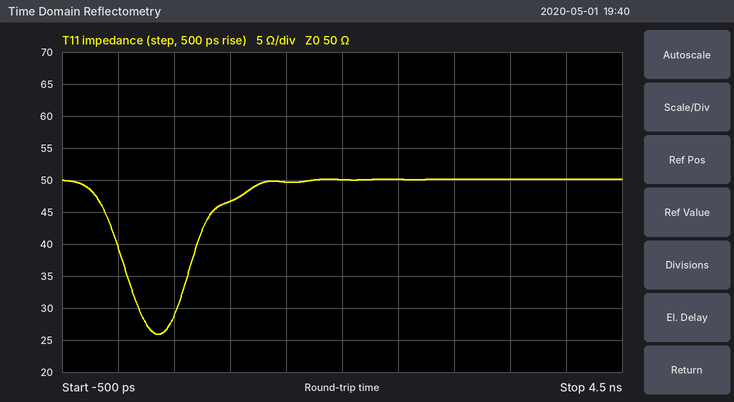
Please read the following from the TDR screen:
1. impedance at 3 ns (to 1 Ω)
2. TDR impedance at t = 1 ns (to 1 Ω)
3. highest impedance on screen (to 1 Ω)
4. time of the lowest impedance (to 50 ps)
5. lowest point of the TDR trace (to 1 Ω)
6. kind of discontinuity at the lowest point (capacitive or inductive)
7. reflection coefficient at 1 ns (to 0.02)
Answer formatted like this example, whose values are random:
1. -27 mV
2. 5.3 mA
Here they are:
1. 50 Ω
2. 47 Ω
3. 50 Ω
4. 350 ps
5. 26 Ω
6. capacitive
7. -0.04
